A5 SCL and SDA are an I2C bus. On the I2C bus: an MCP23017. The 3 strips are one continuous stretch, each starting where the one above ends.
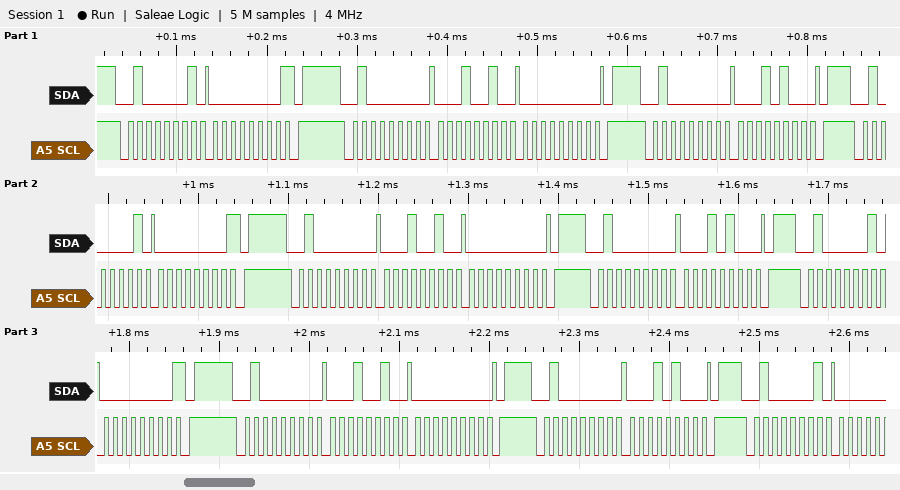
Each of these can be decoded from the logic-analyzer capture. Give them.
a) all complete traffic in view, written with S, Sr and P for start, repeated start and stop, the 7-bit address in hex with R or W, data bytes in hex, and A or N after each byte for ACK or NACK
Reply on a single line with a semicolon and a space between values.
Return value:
S 20R A 00 N P S 20W A 12 A 00 A P S 20W A 14 A P S 20R A 00 N P S 20W A 12 A 00 A P S 20W A 14 A P S 20R A 00 N P S 20W A 12 A 00 A P S 20W A 14 A P S 20R A
